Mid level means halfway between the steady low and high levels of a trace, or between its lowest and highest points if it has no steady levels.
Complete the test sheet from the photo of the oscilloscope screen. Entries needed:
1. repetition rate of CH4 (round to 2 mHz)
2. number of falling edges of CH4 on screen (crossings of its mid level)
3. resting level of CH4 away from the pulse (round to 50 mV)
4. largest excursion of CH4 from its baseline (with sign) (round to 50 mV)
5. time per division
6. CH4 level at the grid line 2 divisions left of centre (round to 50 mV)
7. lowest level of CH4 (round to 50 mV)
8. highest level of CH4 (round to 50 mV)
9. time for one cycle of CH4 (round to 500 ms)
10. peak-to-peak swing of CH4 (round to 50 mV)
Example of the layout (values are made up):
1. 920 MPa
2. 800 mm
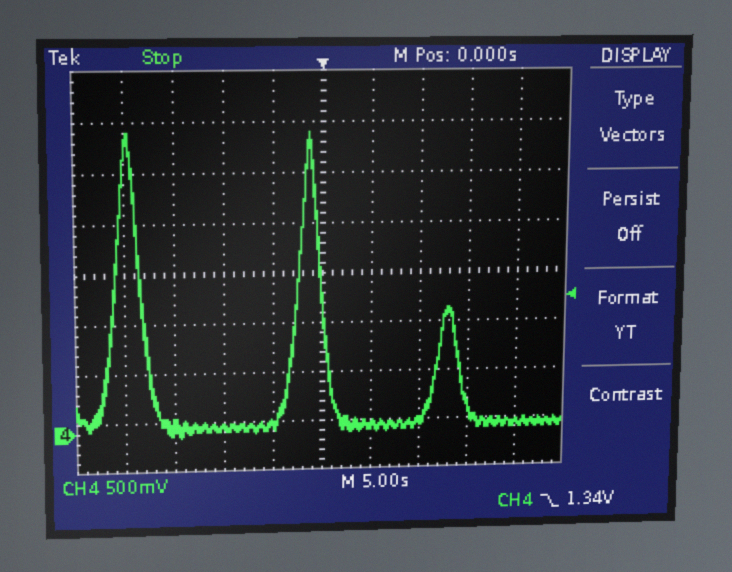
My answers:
1. 54 mHz
2. 2
3. 50 mV
4. +2.95 V
5. 5 s
6. 50 mV
7. -50 mV
8. 3.00 V
9. 18.5 s
10. 3.05 V
